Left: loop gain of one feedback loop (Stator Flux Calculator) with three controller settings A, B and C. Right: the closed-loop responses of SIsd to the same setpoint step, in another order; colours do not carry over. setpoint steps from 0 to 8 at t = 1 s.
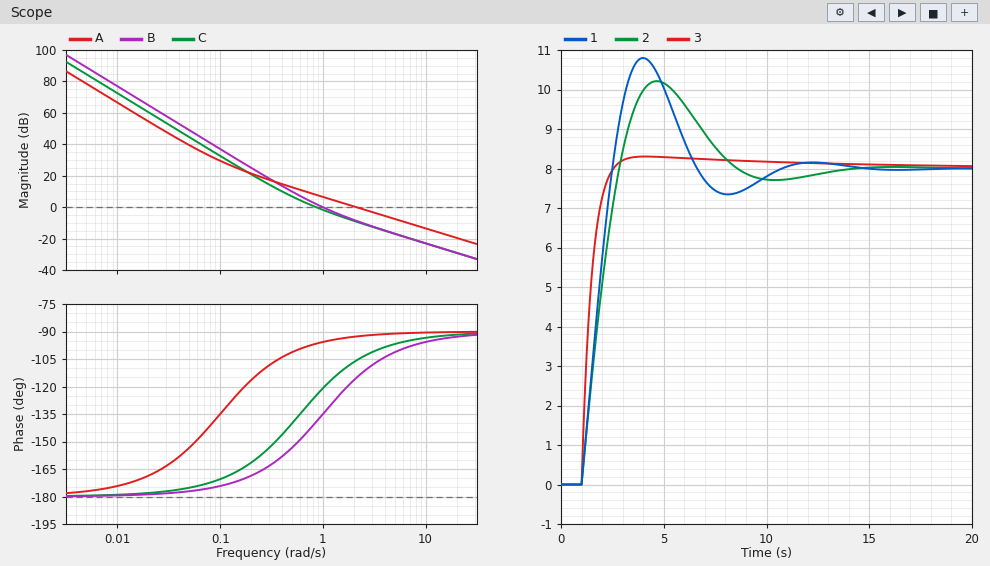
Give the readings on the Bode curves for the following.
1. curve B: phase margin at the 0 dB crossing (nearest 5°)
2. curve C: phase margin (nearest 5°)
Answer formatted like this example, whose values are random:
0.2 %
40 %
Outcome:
45°
55°
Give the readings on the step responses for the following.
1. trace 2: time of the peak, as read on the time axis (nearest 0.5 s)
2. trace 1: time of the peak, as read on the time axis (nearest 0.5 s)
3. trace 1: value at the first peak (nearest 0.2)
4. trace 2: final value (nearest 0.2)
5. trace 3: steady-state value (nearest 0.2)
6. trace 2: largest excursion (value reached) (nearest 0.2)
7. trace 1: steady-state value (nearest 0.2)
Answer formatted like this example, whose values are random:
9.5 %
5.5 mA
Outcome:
4.5 s
4.0 s
10.8
8.0
8.0
10.2
8.0
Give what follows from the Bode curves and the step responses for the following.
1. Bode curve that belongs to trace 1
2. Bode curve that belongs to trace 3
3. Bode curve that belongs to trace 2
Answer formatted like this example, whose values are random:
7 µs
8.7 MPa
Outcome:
B
A
C
